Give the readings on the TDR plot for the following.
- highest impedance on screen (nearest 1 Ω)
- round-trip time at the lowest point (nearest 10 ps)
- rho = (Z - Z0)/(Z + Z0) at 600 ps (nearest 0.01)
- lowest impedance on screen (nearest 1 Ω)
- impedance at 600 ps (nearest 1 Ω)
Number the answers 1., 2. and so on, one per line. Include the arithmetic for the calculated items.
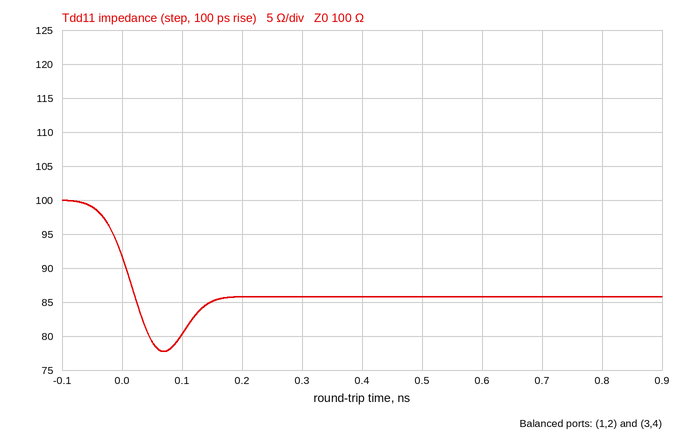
1. 100 Ω
2. 70 ps
3. (86 − 100)/(86 + 100) ≈ -0.08
4. 78 Ω
5. 86 Ω
